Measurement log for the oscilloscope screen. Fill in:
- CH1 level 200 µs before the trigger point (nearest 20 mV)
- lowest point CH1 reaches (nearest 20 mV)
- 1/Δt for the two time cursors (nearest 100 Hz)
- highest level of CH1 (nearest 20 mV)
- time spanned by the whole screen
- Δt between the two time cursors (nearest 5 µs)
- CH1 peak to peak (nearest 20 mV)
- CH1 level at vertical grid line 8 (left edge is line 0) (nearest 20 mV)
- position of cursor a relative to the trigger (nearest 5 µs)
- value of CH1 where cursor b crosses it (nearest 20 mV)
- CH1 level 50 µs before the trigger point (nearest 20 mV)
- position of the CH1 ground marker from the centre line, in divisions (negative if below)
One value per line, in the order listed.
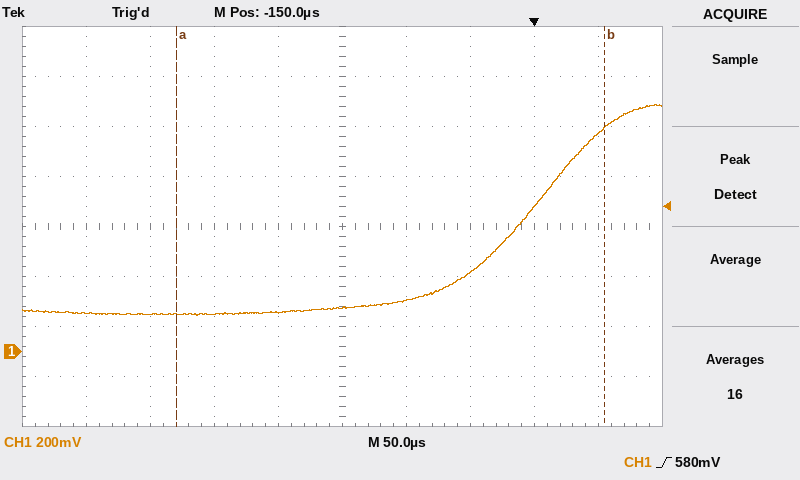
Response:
160 mV
140 mV
3.0 kHz
980 mV
500 µs
335 µs
840 mV
580 mV
-280 µs
900 mV
320 mV
-2.5 div
